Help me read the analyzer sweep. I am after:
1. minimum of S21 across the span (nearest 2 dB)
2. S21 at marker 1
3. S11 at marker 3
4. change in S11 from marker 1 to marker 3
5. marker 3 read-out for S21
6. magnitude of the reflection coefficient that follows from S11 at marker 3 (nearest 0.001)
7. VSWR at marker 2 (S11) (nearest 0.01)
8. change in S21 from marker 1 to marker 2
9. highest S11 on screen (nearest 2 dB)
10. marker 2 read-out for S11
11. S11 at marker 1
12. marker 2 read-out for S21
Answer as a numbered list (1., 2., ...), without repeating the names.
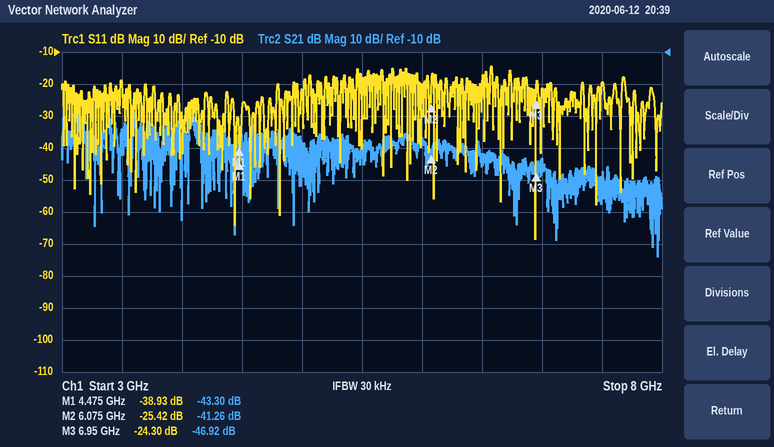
1. -74 dB
2. -43.30 dB
3. -24.30 dB
4. 14.63 dB
5. -46.92 dB
6. 0.061
7. 1.11
8. 2.04 dB
9. -14 dB
10. -25.42 dB
11. -38.93 dB
12. -41.26 dB
